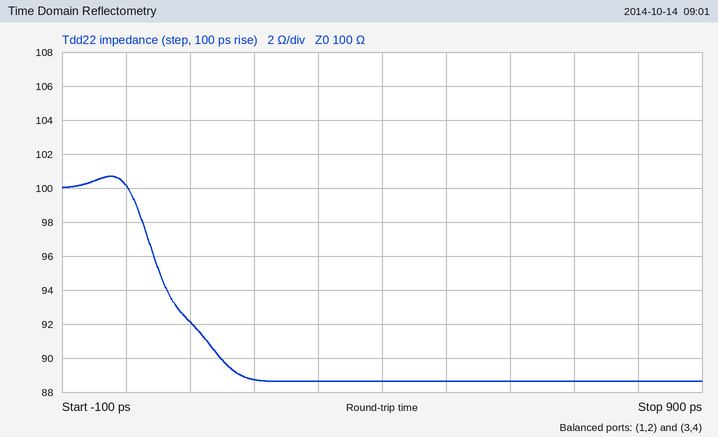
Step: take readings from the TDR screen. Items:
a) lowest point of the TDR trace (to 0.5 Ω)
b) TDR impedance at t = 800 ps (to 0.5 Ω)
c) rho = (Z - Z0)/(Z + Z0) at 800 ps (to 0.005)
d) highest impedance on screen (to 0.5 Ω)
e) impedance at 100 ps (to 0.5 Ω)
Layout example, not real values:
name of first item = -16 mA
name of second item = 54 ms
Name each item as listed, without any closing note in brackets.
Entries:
lowest point of the TDR trace = 88.5 Ω
TDR impedance at t = 800 ps = 88.5 Ω
rho = (Z - Z0)/(Z + Z0) at 800 ps = -0.060
highest impedance on screen = 100.5 Ω
impedance at 100 ps = 92.0 Ω
